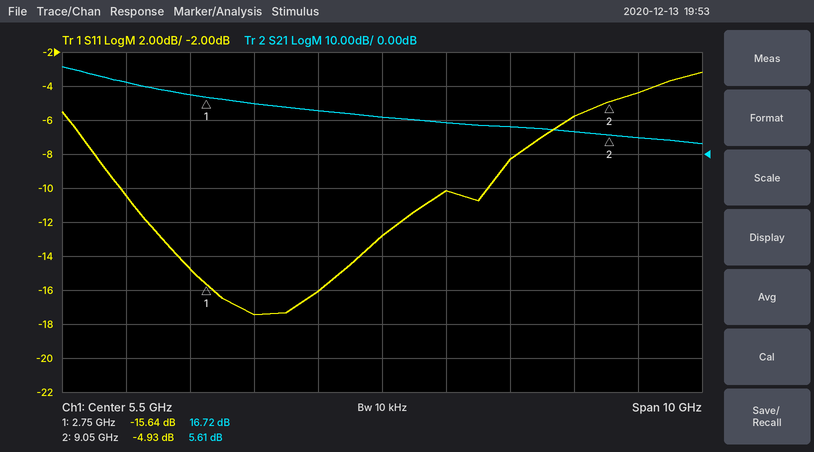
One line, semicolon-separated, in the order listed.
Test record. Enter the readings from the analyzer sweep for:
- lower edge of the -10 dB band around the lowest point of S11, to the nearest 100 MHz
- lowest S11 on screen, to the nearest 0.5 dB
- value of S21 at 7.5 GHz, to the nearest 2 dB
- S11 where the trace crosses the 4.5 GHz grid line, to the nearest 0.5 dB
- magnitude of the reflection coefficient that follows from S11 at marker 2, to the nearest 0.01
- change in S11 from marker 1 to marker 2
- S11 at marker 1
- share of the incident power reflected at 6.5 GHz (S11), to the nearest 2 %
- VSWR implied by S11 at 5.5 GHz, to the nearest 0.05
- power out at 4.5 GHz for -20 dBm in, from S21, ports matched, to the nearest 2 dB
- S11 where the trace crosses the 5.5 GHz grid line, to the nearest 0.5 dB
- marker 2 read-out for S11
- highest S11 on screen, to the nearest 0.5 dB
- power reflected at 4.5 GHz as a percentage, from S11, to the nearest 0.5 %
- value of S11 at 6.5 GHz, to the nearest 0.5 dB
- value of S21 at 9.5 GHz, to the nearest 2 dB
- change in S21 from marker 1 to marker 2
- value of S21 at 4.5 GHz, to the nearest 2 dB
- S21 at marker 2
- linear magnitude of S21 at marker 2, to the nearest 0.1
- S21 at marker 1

1.4 GHz; -17.5 dB; 8 dB; -16.0 dB; 0.57; 10.71 dB; -15.64 dB; 10 %; 1.60; -8 dBm; -13.0 dB; -4.93 dB; -3.0 dB; 2.5 %; -10.0 dB; 4 dB; -11.11 dB; 12 dB; 5.61 dB; 1.9; 16.72 dB
